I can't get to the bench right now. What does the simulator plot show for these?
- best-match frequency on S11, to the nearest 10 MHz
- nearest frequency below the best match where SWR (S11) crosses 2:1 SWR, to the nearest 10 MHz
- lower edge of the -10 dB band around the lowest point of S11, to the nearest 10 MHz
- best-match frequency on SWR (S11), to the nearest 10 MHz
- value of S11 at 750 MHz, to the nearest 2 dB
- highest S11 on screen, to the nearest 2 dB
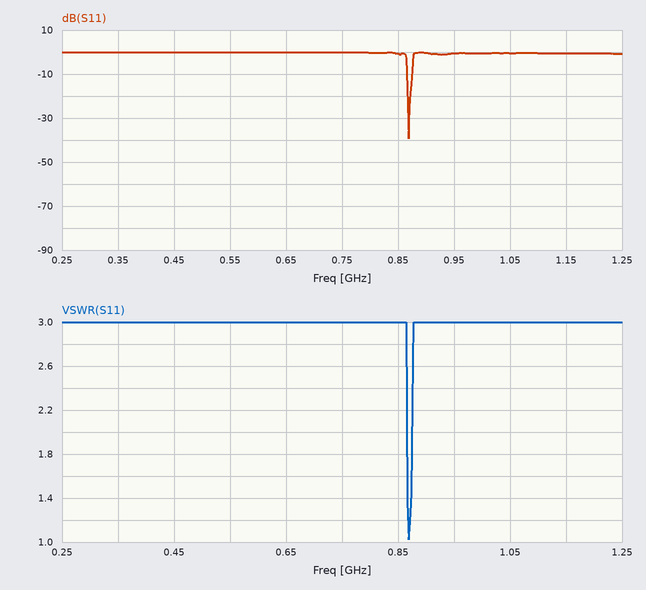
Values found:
870 MHz
870 MHz
870 MHz
870 MHz
0 dB
0 dB
